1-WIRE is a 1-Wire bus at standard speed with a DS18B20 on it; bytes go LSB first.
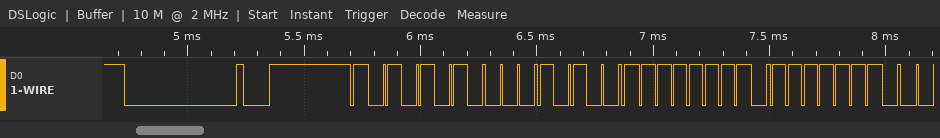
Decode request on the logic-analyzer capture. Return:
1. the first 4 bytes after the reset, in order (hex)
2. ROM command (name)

55 28 FF FE
Match ROM
